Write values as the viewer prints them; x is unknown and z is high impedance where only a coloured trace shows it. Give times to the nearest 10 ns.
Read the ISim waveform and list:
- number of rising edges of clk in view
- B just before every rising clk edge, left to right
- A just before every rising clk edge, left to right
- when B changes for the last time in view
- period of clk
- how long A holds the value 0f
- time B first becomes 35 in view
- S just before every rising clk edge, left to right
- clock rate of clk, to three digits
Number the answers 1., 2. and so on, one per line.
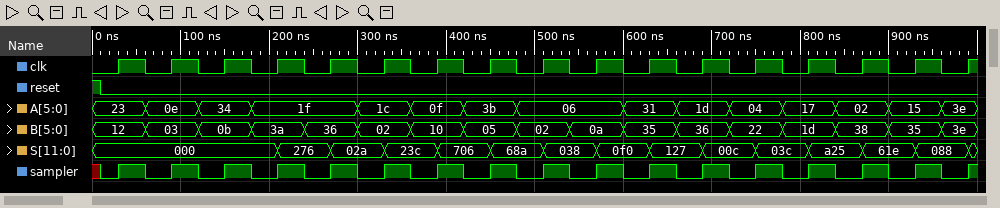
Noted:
1. 17
2. 12, 03, 0b, 3a, 36, 02, 10, 05, 02, 0a, 35, 36, 22, 1d, 38, 35, 3e
3. 23, 0e, 34, 1f, 1f, 1c, 0f, 3b, 06, 06, 31, 1d, 04, 17, 02, 15, 3e
4. 960 ns
5. 60 ns
6. 60 ns
7. 600 ns
8. 000, 000, 000, 000, 276, 02a, 23c, 706, 68a, 038, 0f0, 127, 00c, 03c, a25, 61e, 088
9. 16.7 MHz
